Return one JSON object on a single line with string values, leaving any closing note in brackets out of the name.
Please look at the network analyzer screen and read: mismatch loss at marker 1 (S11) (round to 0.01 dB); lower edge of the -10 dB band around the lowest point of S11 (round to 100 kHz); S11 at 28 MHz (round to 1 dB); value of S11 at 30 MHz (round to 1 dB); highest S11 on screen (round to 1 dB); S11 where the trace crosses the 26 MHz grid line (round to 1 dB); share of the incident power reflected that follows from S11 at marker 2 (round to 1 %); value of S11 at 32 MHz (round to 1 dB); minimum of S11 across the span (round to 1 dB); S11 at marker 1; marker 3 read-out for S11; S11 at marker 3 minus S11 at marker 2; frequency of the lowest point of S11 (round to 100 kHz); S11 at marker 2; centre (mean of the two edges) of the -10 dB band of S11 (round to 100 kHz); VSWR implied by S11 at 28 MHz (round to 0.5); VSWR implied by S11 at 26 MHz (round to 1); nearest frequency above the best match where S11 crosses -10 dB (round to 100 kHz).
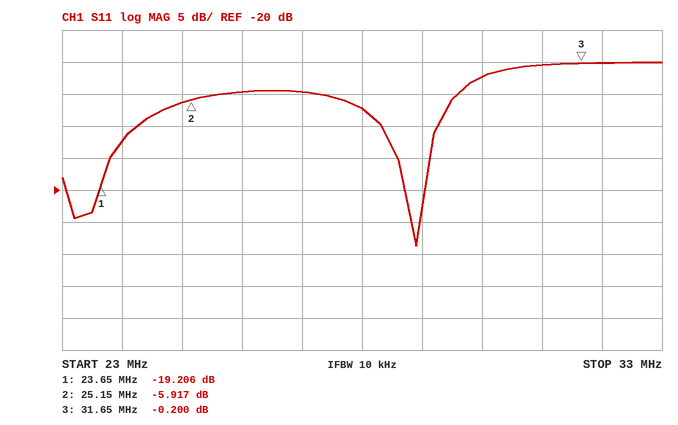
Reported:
{"mismatch loss at marker 1 (S11)": "0.05 dB", "lower edge of the -10 dB band around the lowest point of S11": "28.3 MHz", "S11 at 28 MHz": "-7 dB", "value of S11 at 30 MHz": "-2 dB", "highest S11 on screen": "0 dB", "S11 where the trace crosses the 26 MHz grid line": "-5 dB", "share of the incident power reflected that follows from S11 at marker 2": "26 %", "value of S11 at 32 MHz": "0 dB", "minimum of S11 across the span": "-29 dB", "S11 at marker 1": "-19.206 dB", "marker 3 read-out for S11": "-0.200 dB", "S11 at marker 3 minus S11 at marker 2": "5.717 dB", "frequency of the lowest point of S11": "28.9 MHz", "S11 at marker 2": "-5.917 dB", "centre (mean of the two edges) of the -10 dB band of S11": "28.8 MHz", "VSWR implied by S11 at 28 MHz": "2.5", "VSWR implied by S11 at 26 MHz": "4", "nearest frequency above the best match where S11 crosses -10 dB": "29.3 MHz"}
